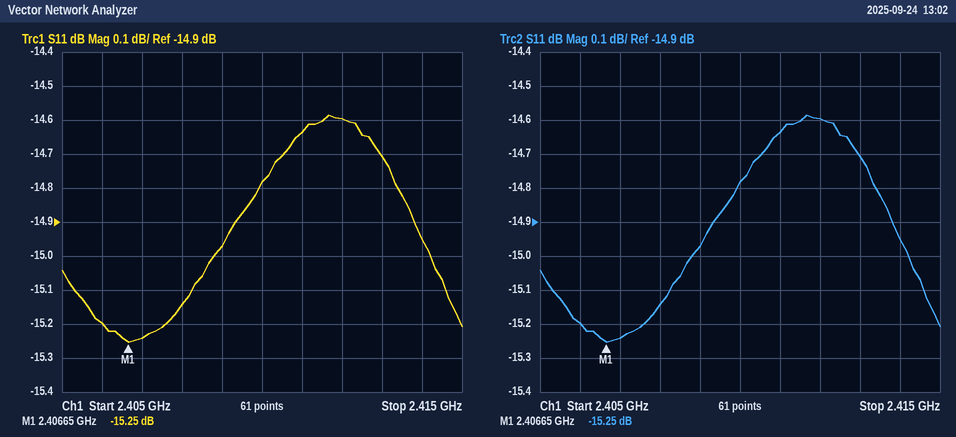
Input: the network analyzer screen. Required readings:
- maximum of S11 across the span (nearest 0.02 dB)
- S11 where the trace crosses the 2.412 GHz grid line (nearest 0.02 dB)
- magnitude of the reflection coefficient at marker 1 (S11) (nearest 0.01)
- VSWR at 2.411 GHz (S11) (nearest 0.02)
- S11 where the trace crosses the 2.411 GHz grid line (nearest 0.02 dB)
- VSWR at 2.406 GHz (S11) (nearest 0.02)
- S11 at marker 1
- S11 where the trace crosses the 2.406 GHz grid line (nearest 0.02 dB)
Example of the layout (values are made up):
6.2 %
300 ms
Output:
-14.58 dB
-14.60 dB
0.17
1.46
-14.64 dB
1.42
-15.25 dB
-15.20 dB
